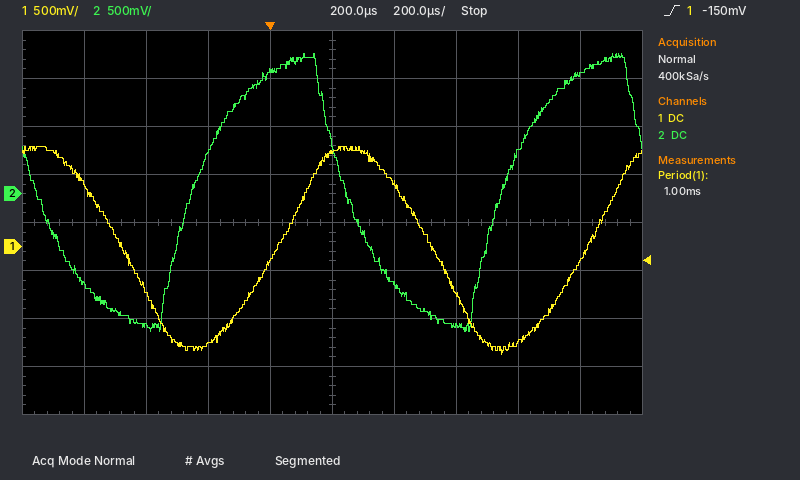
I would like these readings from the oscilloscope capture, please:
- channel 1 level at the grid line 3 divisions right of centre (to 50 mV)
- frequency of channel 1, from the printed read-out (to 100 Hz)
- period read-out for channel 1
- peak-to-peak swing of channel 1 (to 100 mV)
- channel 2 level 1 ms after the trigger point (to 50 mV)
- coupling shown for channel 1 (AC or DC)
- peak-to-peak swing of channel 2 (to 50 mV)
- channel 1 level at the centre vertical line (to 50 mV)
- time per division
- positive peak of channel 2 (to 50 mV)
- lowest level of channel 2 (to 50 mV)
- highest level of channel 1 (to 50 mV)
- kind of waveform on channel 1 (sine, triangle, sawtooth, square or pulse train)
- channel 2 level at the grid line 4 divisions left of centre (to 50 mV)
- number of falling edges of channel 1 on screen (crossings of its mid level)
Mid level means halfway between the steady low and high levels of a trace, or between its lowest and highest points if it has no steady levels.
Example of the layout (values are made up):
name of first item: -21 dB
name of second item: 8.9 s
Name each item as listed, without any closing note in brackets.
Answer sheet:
channel 1 level at the grid line 3 divisions right of centre: -1.00 V
frequency of channel 1, from the printed read-out: 1.0 kHz
period read-out for channel 1: 1.00 ms
peak-to-peak swing of channel 1: 2.20 V
channel 2 level 1 ms after the trigger point: 1.25 V
coupling shown for channel 1: DC
peak-to-peak swing of channel 2: 2.90 V
channel 1 level at the centre vertical line: 1.00 V
time per division: 200 µs
positive peak of channel 2: 1.45 V
lowest level of channel 2: -1.45 V
highest level of channel 1: 1.05 V
kind of waveform on channel 1: sine
channel 2 level at the grid line 4 divisions left of centre: -950 mV
number of falling edges of channel 1 on screen: 2
